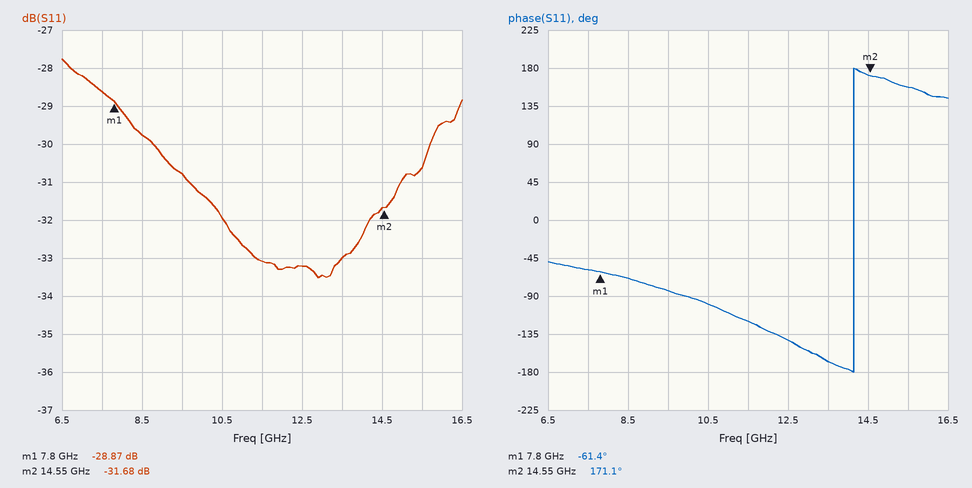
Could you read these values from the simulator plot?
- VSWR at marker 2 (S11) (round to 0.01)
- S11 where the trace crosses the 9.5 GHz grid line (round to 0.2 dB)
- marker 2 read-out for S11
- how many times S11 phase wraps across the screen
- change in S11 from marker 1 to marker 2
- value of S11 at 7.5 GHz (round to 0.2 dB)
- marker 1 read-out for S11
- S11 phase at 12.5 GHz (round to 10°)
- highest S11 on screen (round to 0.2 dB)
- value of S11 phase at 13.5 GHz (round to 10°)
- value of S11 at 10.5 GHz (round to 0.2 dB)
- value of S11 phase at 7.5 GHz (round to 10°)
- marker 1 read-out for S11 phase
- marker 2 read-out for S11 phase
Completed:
1.05
-30.8 dB
-31.68 dB
1
-2.81 dB
-28.6 dB
-28.87 dB
-140°
-27.8 dB
-170°
-32.0 dB
-60°
-61.4°
171.1°
